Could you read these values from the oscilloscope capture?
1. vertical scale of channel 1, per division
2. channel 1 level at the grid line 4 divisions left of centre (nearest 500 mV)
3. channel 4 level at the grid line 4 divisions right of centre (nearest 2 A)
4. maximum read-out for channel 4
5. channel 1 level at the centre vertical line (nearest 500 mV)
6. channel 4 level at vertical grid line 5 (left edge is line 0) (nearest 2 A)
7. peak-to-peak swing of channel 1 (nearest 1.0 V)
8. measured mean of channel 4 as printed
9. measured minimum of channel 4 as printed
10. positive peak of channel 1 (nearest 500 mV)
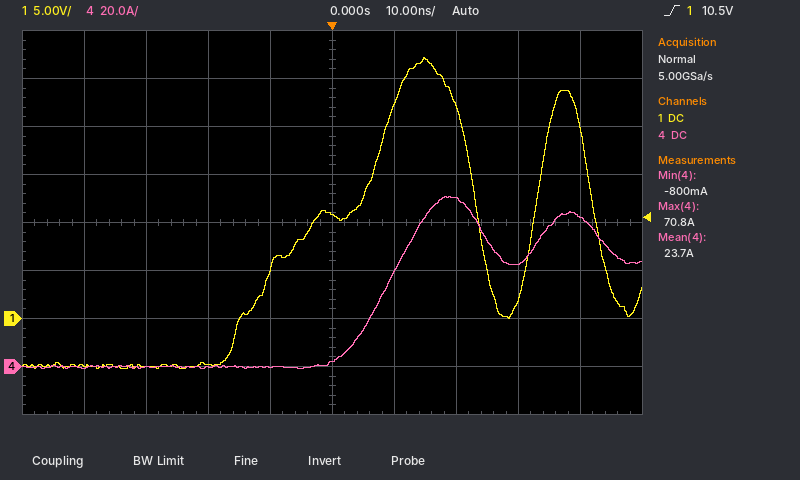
5 V
-5.0 V
62 A
70.8 A
11.0 V
2 A
32.0 V
23.7 A
-800 mA
27.0 V
